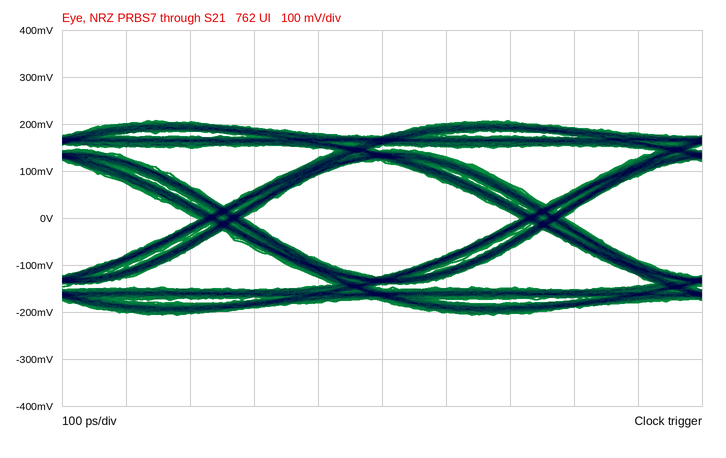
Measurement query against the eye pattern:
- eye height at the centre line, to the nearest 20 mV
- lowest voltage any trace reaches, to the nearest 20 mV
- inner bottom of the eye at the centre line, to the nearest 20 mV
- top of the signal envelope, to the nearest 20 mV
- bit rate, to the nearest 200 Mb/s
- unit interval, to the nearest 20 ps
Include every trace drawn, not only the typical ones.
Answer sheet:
240 mV
-200 mV
-120 mV
200 mV
2.0 Gb/s
500 ps
